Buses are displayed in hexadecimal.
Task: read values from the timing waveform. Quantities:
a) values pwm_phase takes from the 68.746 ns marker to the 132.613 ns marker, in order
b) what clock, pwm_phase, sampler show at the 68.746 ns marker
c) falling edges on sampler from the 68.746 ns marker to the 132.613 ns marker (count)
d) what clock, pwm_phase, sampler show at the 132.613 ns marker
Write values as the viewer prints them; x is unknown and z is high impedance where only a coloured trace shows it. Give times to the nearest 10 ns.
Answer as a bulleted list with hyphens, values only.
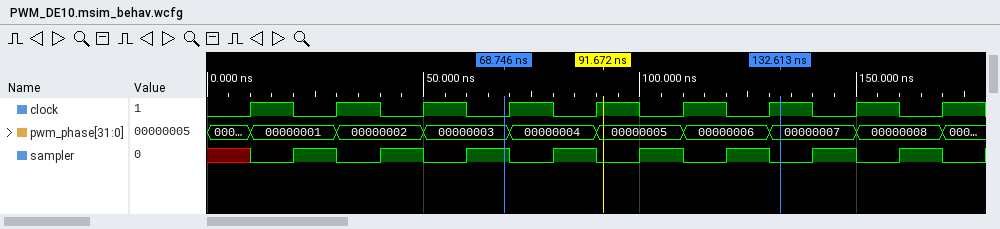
- 00000003, 00000004, 00000005, 00000006, 00000007
- clock=0, pwm_phase=00000003, sampler=1
- 4
- clock=1, pwm_phase=00000007, sampler=0
